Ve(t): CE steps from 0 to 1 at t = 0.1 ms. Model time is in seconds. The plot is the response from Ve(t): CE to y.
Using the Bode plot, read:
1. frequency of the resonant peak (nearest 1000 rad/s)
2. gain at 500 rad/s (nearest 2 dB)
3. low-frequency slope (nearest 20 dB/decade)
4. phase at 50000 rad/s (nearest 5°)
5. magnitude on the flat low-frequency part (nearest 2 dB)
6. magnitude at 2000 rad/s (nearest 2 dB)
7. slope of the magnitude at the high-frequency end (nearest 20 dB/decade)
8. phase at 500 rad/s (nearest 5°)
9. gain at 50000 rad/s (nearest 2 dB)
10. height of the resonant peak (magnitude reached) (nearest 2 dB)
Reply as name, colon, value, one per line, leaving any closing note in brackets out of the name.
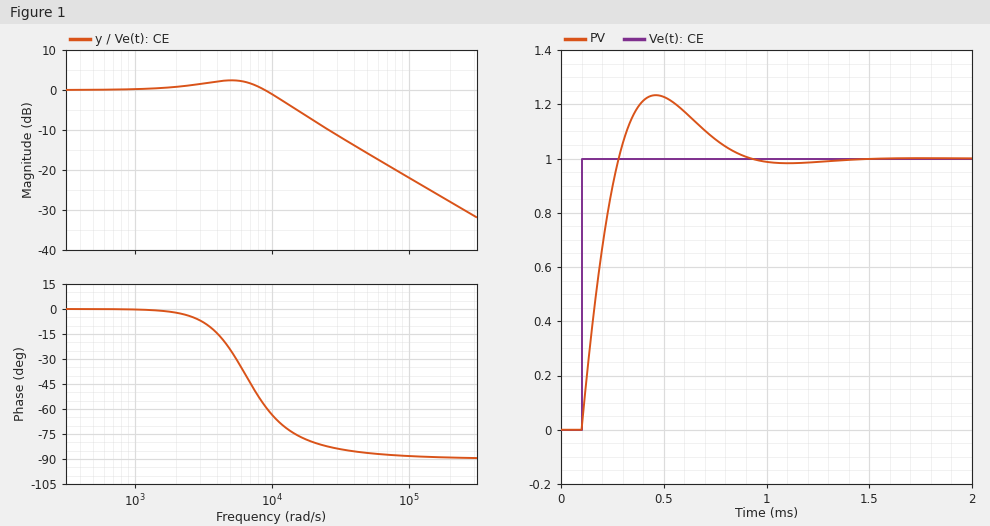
frequency of the resonant peak: 5000 rad/s
gain at 500 rad/s: 0 dB
low-frequency slope: 0 dB/decade
phase at 50000 rad/s: -85°
magnitude on the flat low-frequency part: 0 dB
magnitude at 2000 rad/s: 0 dB
slope of the magnitude at the high-frequency end: -20 dB/decade
phase at 500 rad/s: 0°
gain at 50000 rad/s: -16 dB
height of the resonant peak (magnitude reached): 2 dB
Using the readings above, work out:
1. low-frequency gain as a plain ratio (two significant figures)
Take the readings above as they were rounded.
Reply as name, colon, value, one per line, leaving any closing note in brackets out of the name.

low-frequency gain as a plain ratio: 1.0
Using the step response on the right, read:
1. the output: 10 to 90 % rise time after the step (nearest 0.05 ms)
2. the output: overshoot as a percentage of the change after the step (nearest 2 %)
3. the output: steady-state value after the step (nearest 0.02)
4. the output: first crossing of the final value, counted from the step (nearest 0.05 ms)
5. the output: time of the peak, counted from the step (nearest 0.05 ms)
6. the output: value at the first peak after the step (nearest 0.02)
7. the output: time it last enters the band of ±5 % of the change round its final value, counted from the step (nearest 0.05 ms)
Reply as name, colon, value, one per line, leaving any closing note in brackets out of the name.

the output: 10 to 90 % rise time after the step: 0.15 ms
the output: overshoot as a percentage of the change after the step: 24 %
the output: steady-state value after the step: 1.00
the output: first crossing of the final value, counted from the step: 0.20 ms
the output: time of the peak, counted from the step: 0.35 ms
the output: value at the first peak after the step: 1.24
the output: time it last enters the band of ±5 % of the change round its final value, counted from the step: 0.70 ms
